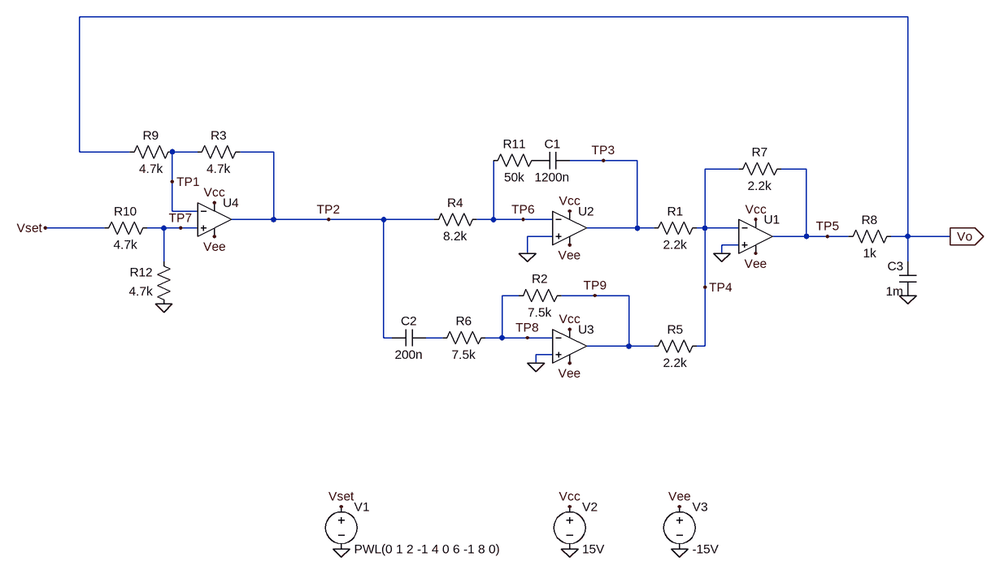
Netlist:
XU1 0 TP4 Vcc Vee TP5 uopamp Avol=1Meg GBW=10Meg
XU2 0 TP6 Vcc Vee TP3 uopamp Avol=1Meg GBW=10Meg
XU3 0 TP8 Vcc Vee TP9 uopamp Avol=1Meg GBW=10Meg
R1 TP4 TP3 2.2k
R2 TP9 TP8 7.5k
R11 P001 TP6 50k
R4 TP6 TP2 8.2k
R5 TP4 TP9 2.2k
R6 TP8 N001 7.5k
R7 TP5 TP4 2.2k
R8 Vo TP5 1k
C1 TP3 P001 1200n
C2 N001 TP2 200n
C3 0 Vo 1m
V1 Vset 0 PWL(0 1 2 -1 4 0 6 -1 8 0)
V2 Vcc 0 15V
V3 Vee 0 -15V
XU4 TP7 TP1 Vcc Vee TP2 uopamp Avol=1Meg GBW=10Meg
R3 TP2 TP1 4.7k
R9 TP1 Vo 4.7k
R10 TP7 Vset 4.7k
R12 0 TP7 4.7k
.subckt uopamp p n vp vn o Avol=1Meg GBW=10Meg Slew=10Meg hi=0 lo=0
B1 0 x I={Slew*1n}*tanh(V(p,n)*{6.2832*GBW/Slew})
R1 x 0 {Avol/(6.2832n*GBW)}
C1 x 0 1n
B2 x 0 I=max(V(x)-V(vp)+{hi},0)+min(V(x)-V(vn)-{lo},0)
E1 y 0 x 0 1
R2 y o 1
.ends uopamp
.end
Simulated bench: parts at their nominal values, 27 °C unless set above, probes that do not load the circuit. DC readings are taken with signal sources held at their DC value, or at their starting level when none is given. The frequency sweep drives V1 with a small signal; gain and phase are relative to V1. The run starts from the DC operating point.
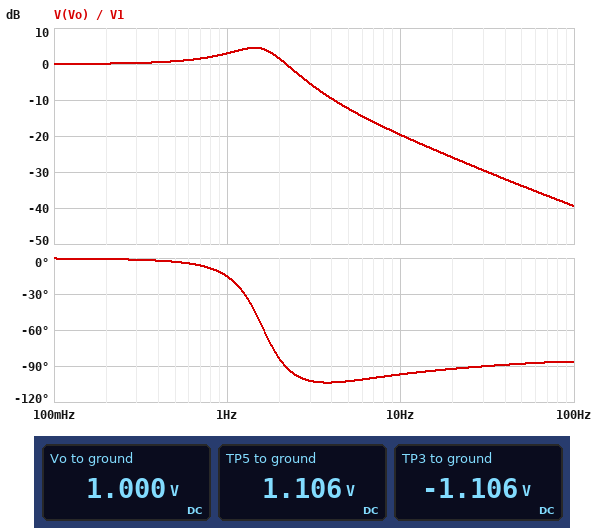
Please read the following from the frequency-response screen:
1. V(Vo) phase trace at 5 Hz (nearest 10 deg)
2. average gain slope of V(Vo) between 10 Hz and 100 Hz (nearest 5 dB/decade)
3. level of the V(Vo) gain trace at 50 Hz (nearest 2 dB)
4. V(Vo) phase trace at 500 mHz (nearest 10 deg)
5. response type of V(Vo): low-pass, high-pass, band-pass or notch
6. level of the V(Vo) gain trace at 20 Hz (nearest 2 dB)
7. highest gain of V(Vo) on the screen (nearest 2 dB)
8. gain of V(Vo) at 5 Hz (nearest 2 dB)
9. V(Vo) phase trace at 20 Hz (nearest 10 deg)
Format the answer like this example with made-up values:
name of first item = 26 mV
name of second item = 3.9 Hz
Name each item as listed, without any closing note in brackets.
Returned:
V(Vo) phase trace at 5 Hz = -100 deg
average gain slope of V(Vo) between 10 Hz and 100 Hz = -20 dB/decade
level of the V(Vo) gain trace at 50 Hz = -34 dB
V(Vo) phase trace at 500 mHz = 0 deg
response type of V(Vo): low-pass, high-pass, band-pass or notch = low-pass
level of the V(Vo) gain trace at 20 Hz = -26 dB
highest gain of V(Vo) on the screen = 4 dB
gain of V(Vo) at 5 Hz = -12 dB
V(Vo) phase trace at 20 Hz = -90 deg
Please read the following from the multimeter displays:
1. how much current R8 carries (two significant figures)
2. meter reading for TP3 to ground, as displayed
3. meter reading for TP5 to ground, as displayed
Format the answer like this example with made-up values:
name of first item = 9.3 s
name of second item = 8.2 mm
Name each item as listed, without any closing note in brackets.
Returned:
how much current R8 carries = 110 µA
meter reading for TP3 to ground, as displayed = -1.106 V
meter reading for TP5 to ground, as displayed = 1.106 V
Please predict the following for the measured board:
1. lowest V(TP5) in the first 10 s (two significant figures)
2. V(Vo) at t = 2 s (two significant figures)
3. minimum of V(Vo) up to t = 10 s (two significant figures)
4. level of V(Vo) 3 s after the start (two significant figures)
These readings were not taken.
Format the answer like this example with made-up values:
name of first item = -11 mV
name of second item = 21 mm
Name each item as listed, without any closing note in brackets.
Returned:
lowest V(TP5) in the first 10 s = -2.1 V
V(Vo) at t = 2 s = -990 mV
minimum of V(Vo) up to t = 10 s = -1.0 V
level of V(Vo) 3 s after the start = -510 mV
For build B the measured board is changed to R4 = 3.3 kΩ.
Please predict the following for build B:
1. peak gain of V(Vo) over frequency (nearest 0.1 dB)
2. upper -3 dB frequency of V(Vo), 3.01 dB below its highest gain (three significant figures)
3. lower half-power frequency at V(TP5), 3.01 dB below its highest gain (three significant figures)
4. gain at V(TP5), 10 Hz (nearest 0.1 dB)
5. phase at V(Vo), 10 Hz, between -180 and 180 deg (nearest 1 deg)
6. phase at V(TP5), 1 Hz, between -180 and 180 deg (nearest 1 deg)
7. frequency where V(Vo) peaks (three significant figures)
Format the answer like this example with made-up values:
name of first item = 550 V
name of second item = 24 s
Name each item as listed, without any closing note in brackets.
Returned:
peak gain of V(Vo) over frequency = 3.0 dB
upper -3 dB frequency of V(Vo), 3.01 dB below its highest gain = 3.46 Hz
lower half-power frequency at V(TP5), 3.01 dB below its highest gain = 1.81 Hz
gain at V(TP5), 10 Hz = 24.1 dB
phase at V(Vo), 10 Hz, between -180 and 180 deg = -89 deg
phase at V(TP5), 1 Hz, between -180 and 180 deg = 75 deg
frequency where V(Vo) peaks = 2.12 Hz
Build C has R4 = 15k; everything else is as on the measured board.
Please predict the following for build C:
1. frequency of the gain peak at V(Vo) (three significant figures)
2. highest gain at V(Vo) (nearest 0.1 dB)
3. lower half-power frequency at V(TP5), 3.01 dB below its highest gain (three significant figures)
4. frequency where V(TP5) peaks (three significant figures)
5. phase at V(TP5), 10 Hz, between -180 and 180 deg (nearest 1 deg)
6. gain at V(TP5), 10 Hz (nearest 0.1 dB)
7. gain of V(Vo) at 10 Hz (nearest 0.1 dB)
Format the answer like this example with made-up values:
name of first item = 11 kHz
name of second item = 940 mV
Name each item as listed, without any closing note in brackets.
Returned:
frequency of the gain peak at V(Vo) = 1.09 Hz
highest gain at V(Vo) = 5.4 dB
lower half-power frequency at V(TP5), 3.01 dB below its highest gain = 893 mHz
frequency where V(TP5) peaks = 1.20 Hz
phase at V(TP5), 10 Hz, between -180 and 180 deg = -10 deg
gain at V(TP5), 10 Hz = 10.8 dB
gain of V(Vo) at 10 Hz = -24.9 dB
